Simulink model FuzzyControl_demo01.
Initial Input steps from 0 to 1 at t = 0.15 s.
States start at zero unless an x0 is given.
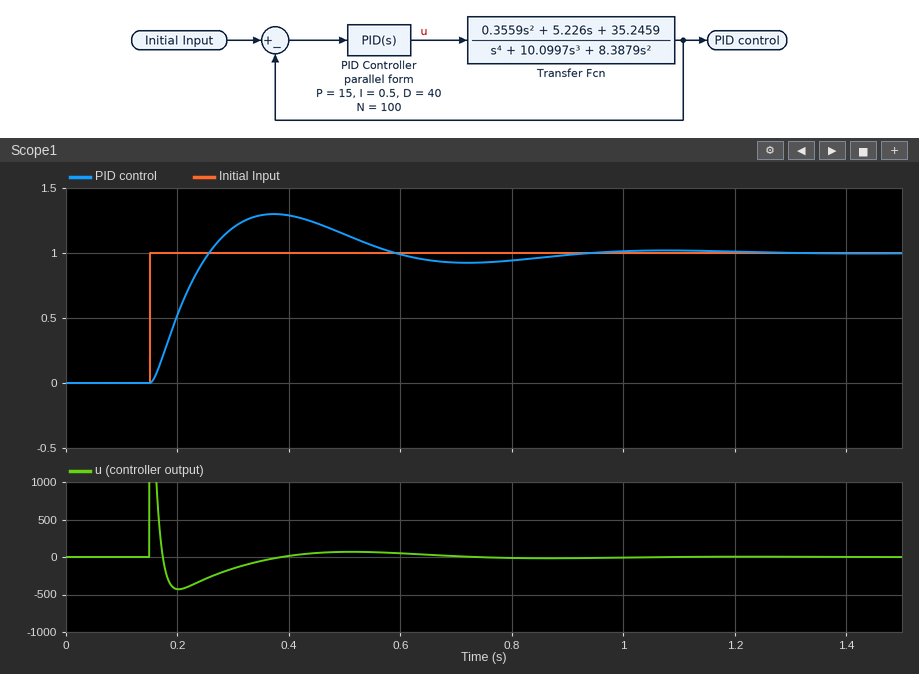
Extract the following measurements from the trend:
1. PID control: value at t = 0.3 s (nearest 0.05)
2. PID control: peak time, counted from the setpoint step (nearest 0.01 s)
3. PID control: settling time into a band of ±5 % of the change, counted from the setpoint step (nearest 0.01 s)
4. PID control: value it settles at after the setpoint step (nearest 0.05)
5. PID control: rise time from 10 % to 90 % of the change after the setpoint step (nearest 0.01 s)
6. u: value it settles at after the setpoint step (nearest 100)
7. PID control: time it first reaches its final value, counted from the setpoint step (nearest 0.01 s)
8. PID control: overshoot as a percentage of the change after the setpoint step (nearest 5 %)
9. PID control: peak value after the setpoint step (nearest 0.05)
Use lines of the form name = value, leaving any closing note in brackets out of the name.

PID control: value at t = 0.3 s = 1.20
PID control: peak time, counted from the setpoint step = 0.22 s
PID control: settling time into a band of ±5 % of the change, counted from the setpoint step = 0.67 s
PID control: value it settles at after the setpoint step = 1.00
PID control: rise time from 10 % to 90 % of the change after the setpoint step = 0.08 s
u: value it settles at after the setpoint step = 0
PID control: time it first reaches its final value, counted from the setpoint step = 0.11 s
PID control: overshoot as a percentage of the change after the setpoint step = 30 %
PID control: peak value after the setpoint step = 1.30
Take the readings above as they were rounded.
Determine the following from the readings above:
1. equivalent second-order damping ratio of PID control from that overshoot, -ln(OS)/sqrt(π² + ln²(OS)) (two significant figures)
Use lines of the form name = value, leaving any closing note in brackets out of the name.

equivalent second-order damping ratio of PID control from that overshoot, -ln(OS)/sqrt(π² + ln²(OS)) = 0.36
